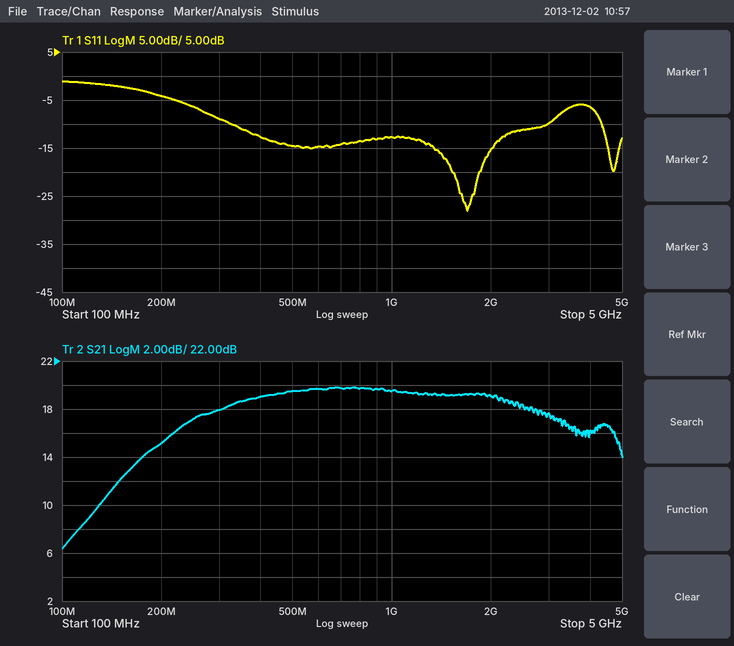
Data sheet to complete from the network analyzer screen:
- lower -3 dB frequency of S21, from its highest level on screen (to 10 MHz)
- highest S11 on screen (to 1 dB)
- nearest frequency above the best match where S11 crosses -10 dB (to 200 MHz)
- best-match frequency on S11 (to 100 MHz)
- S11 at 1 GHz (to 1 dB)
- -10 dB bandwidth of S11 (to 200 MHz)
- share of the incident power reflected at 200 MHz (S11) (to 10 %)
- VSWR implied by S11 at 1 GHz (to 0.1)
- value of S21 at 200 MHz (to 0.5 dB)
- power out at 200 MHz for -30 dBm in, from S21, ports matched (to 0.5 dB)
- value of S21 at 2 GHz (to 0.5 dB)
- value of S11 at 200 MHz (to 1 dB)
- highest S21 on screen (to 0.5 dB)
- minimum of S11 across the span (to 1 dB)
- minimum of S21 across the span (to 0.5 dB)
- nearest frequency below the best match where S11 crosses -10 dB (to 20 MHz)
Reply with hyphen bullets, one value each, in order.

- 240 MHz
- -1 dB
- 3.0 GHz
- 1.7 GHz
- -13 dB
- 2.6 GHz
- 40 %
- 1.6
- 15.0 dB
- -15.0 dBm
- 19.0 dB
- -4 dB
- 20.0 dB
- -28 dB
- 6.5 dB
- 320 MHz
